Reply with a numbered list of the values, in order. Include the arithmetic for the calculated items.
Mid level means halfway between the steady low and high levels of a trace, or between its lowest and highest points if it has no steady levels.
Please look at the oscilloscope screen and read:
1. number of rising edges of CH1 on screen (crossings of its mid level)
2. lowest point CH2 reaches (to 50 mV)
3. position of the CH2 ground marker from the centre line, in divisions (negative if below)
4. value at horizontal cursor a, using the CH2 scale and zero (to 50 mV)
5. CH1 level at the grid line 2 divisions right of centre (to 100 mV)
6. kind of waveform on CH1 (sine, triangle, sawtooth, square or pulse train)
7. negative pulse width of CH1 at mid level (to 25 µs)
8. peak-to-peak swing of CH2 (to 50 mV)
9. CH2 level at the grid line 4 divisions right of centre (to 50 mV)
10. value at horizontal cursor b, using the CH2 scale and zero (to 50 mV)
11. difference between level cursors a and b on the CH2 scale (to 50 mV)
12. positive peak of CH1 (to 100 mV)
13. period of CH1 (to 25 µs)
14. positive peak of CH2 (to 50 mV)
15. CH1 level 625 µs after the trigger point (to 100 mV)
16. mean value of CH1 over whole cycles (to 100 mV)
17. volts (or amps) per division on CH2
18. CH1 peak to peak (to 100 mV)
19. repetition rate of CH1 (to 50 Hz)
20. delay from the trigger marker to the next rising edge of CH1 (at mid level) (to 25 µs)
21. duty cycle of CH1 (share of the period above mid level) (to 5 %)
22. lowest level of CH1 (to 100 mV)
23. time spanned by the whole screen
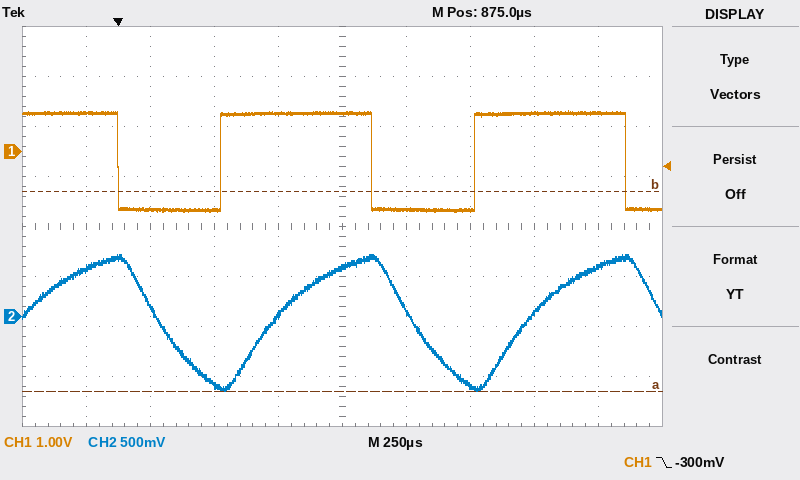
1. 2
2. -750 mV
3. -1.8 div
4. -750 mV
5. -1.2 V
6. pulse train
7. 400 µs
8. 600 mV − (-750 mV) = 1.35 V
9. 500 mV
10. 1.25 V
11. 2.00 V
12. 800 mV
13. 1.000 ms
14. 600 mV
15. 800 mV
16. -1.2 V + 0.6 × (800 mV − (-1.2 V)) ≈ 0.0 V
17. 500 mV
18. 800 mV − (-1.2 V) = 2.0 V
19. 1 / 1.000 ms ≈ 1.00 kHz
20. 400 µs
21. 60 %
22. -1.2 V
23. 2.5 ms
